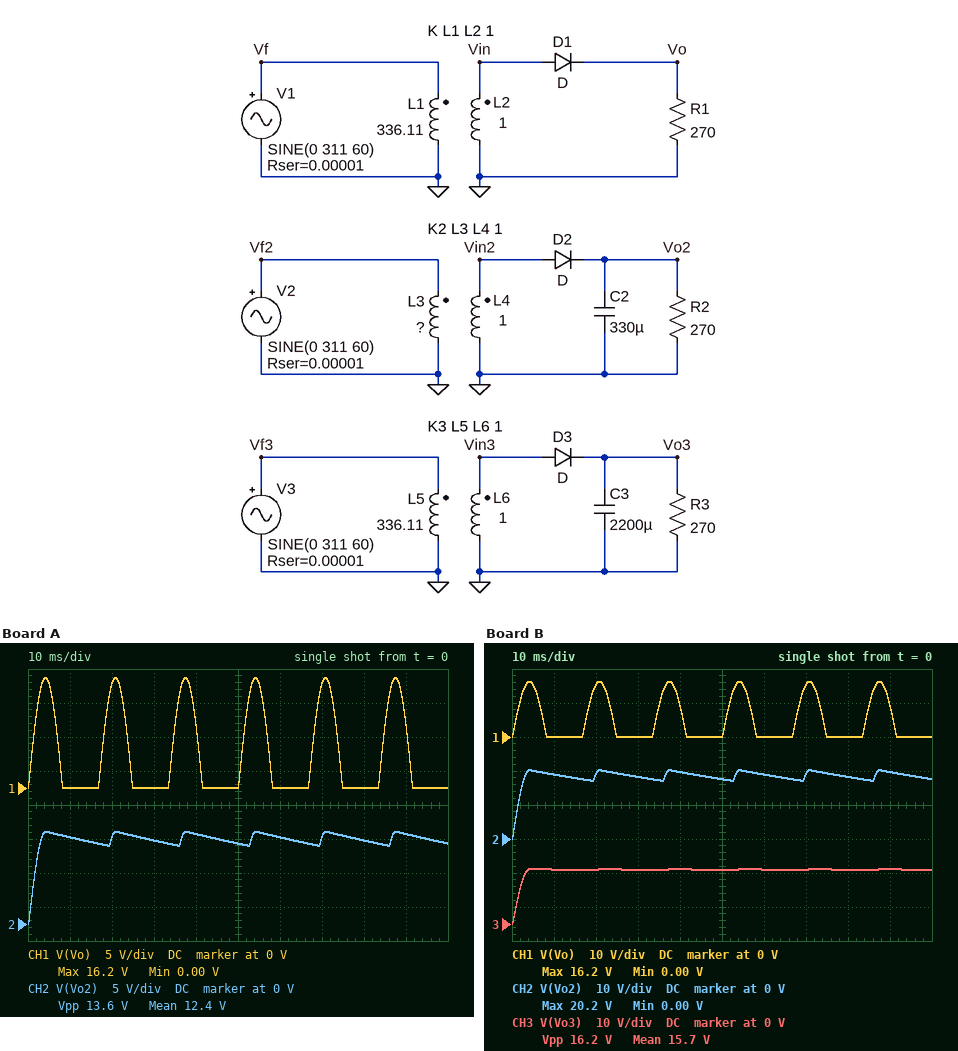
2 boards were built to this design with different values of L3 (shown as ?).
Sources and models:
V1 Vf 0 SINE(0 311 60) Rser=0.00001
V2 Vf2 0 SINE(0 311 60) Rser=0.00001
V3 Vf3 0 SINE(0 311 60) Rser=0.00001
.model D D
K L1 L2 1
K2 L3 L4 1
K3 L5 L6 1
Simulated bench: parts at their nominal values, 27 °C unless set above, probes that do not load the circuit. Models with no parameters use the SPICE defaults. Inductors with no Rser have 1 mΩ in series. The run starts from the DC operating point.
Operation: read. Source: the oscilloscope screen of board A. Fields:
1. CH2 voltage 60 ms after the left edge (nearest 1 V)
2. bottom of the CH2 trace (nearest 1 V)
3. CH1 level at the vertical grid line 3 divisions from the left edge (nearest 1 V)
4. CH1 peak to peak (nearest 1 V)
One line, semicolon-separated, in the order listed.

13 V; 0 V; 0 V; 16 V
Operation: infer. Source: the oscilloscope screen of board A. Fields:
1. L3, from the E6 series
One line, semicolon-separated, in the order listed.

470 H
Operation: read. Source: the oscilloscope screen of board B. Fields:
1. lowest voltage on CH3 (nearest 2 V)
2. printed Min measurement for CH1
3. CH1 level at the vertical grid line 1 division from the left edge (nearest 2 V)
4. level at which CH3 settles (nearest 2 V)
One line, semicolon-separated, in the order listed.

0 V; 0.00 V; 0 V; 16 V
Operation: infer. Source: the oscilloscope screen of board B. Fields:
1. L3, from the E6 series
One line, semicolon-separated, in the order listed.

220 H
